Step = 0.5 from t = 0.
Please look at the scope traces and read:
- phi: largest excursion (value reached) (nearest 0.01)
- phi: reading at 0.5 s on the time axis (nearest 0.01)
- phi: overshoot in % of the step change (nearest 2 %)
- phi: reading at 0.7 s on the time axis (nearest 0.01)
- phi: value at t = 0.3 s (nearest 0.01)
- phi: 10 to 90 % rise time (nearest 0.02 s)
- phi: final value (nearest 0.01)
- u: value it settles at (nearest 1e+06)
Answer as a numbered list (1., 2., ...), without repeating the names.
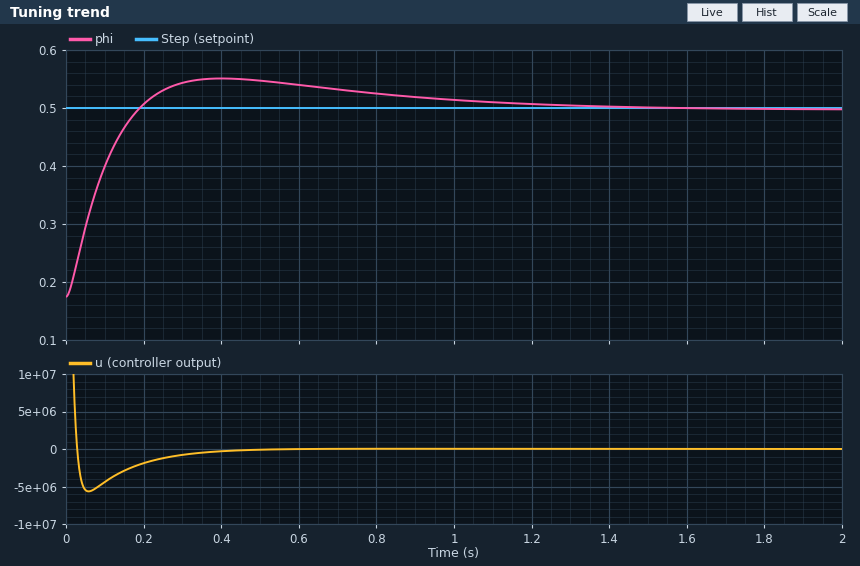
1. 0.55
2. 0.55
3. 16 %
4. 0.53
5. 0.54
6. 0.14 s
7. 0.50
8. 0
